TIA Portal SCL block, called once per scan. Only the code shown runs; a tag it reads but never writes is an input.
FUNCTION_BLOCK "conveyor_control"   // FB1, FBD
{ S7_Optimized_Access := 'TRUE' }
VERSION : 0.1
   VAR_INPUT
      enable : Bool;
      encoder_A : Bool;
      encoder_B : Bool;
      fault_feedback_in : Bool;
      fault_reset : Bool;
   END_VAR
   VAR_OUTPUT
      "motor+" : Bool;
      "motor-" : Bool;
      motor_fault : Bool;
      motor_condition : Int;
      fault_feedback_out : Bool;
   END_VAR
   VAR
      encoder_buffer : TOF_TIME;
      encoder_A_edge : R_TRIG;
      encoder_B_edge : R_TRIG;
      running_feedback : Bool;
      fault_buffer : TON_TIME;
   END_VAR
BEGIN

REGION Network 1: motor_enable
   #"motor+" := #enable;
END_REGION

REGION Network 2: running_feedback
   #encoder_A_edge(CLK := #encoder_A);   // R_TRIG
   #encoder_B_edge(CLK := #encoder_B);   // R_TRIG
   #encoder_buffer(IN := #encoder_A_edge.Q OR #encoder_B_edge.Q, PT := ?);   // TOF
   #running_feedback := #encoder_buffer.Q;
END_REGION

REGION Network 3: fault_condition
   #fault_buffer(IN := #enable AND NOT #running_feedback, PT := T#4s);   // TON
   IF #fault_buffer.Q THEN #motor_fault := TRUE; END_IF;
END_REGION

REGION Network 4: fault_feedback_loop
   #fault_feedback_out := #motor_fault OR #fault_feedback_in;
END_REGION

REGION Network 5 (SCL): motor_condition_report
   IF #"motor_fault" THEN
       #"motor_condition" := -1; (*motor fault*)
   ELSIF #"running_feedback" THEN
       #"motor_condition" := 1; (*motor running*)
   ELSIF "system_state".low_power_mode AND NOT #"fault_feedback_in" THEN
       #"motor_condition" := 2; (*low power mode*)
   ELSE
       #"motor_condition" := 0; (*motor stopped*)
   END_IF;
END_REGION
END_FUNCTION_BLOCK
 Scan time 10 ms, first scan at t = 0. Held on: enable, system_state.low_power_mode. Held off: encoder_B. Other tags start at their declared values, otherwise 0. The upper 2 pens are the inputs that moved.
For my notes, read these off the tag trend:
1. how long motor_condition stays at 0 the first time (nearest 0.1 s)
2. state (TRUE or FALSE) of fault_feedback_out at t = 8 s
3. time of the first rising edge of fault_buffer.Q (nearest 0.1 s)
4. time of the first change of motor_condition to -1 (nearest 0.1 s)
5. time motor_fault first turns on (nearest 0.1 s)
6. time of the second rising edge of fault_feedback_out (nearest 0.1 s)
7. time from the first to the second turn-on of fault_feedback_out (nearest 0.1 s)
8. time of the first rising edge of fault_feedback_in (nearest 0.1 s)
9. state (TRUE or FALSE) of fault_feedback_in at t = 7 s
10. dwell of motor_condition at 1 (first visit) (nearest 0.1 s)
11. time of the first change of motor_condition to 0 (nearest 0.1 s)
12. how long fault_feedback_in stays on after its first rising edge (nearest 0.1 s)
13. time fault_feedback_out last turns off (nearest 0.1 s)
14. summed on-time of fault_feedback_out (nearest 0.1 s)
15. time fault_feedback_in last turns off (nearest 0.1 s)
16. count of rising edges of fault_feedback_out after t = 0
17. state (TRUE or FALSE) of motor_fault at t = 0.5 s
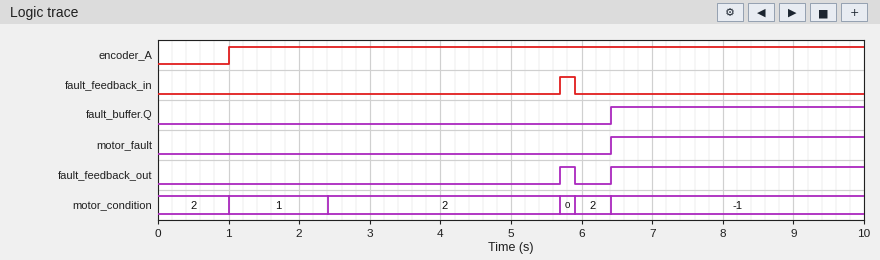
0.2 s
TRUE
6.4 s
6.4 s
6.4 s
6.4 s
0.7 s
5.7 s
FALSE
1.4 s
5.7 s
0.2 s
5.9 s
3.8 s
5.9 s
2
FALSE
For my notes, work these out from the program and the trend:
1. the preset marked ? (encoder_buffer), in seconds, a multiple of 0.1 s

1.4 s
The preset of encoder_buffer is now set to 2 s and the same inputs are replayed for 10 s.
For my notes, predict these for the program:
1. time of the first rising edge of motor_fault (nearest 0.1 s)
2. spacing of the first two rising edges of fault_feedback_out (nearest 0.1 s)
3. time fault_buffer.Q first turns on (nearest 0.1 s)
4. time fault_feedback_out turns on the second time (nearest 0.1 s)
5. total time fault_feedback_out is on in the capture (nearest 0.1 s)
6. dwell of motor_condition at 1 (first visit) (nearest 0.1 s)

7.0 s
1.3 s
7.0 s
7.0 s
3.2 s
2.0 s
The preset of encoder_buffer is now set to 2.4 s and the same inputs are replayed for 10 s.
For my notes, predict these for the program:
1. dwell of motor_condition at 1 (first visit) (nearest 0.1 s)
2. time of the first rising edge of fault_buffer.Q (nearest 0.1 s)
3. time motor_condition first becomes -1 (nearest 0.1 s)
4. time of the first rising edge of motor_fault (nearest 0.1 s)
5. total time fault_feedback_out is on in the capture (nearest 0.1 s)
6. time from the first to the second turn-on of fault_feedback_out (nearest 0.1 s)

2.4 s
7.4 s
7.4 s
7.4 s
2.8 s
1.7 s
